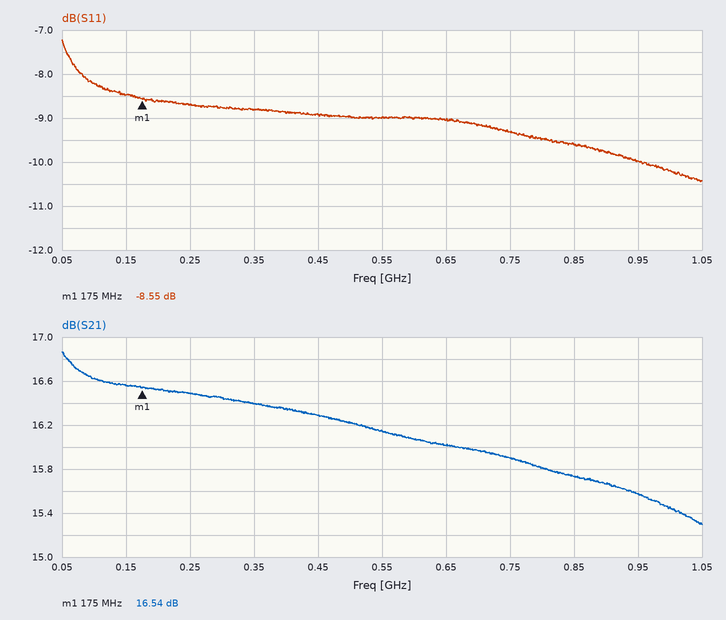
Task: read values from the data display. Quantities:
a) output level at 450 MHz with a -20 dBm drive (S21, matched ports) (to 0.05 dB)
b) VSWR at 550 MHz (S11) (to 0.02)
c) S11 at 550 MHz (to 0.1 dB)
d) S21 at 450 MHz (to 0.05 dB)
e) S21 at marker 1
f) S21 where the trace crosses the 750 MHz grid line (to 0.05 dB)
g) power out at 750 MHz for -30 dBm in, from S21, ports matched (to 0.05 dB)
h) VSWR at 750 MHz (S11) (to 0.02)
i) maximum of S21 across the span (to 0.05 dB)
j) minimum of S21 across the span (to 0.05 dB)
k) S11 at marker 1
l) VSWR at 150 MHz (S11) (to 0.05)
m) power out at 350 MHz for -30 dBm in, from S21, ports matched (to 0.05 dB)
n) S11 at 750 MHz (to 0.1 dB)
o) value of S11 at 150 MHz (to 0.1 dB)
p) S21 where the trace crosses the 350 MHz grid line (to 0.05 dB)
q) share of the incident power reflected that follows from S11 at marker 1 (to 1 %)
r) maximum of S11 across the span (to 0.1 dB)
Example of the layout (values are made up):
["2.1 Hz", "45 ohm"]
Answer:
["-3.70 dBm", "2.10", "-9.0 dB", "16.30 dB", "16.54 dB", "15.90 dB", "-14.10 dBm", "2.04", "16.85 dB", "15.30 dB", "-8.55 dB", "2.20", "-13.60 dBm", "-9.3 dB", "-8.5 dB", "16.40 dB", "14 %", "-7.2 dB"]
